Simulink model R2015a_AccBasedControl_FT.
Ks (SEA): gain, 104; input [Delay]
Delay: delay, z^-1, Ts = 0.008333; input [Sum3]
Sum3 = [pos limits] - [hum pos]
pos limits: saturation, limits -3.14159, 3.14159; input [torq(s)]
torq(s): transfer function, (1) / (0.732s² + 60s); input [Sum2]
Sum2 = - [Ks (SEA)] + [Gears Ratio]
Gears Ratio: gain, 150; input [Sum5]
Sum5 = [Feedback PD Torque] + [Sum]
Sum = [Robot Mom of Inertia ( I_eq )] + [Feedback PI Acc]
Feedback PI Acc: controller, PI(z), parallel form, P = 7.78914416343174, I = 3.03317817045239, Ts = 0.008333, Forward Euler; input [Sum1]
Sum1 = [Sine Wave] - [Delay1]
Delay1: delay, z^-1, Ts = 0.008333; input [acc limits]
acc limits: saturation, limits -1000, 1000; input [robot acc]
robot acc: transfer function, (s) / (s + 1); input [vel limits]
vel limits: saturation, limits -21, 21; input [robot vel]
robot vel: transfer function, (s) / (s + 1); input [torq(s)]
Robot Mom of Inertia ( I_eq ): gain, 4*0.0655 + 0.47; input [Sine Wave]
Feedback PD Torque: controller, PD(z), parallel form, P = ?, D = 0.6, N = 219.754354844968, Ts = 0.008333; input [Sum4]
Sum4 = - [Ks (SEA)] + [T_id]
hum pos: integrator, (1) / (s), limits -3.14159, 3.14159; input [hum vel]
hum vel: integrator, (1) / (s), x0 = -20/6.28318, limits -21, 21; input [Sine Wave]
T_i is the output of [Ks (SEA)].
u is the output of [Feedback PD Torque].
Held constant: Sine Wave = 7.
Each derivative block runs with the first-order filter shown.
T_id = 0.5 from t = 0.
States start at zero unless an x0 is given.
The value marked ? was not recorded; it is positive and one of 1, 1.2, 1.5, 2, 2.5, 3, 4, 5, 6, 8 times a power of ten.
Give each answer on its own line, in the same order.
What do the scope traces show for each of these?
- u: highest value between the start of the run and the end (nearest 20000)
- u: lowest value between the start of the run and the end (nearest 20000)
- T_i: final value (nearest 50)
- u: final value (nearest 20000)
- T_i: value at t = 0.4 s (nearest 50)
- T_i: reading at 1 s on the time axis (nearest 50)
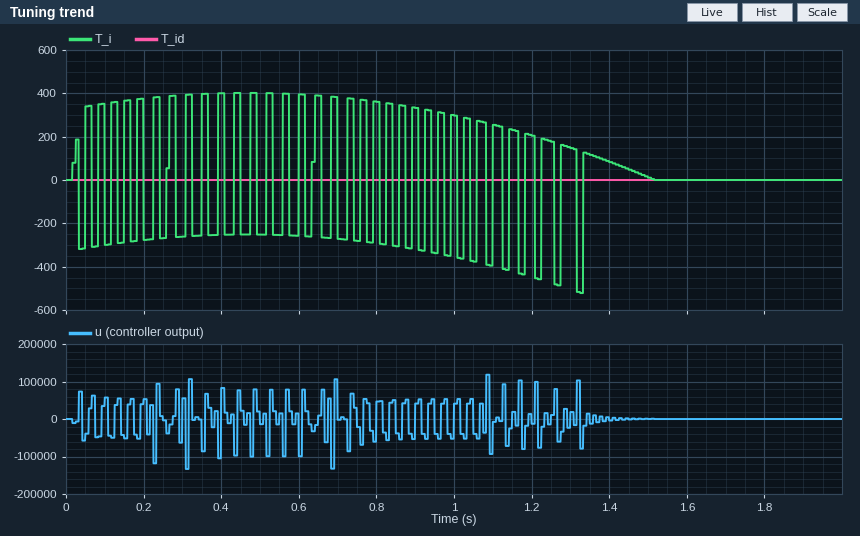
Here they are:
120000
-140000
0
0
400
300
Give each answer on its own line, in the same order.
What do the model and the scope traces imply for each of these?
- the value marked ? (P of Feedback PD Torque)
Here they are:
6
